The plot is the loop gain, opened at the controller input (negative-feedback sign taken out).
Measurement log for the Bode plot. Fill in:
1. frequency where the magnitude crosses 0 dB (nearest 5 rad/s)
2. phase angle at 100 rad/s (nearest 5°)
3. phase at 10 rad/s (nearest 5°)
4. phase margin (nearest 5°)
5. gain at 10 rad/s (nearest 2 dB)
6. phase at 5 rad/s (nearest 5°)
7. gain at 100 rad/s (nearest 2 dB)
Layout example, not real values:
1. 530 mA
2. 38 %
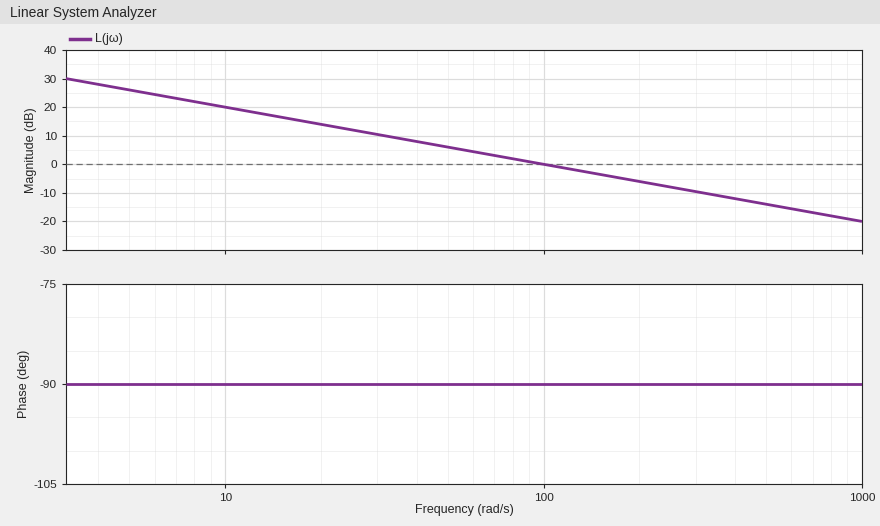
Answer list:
1. 100 rad/s
2. -90°
3. -90°
4. 90°
5. 20 dB
6. -90°
7. 0 dB
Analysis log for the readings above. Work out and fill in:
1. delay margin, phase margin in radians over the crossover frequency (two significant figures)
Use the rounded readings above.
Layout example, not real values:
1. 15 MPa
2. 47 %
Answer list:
1. 0.016 s
